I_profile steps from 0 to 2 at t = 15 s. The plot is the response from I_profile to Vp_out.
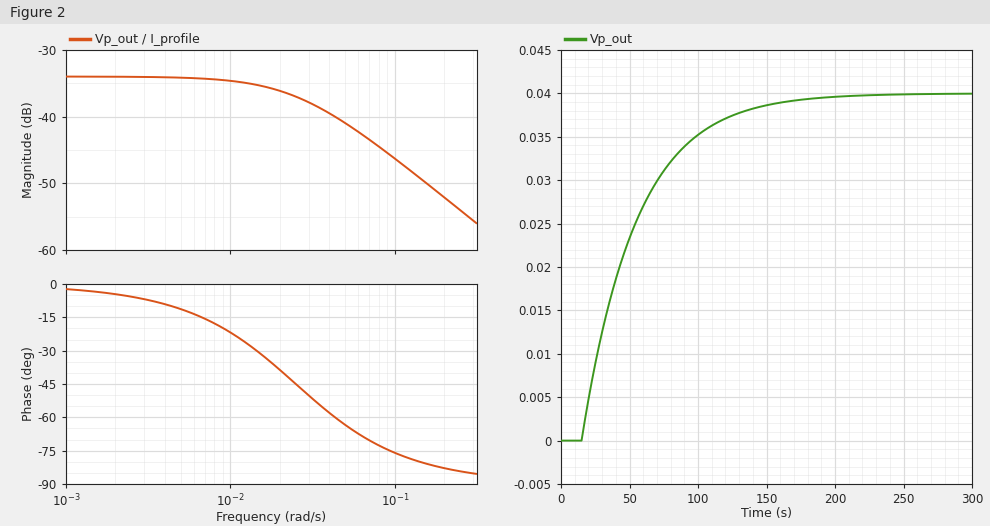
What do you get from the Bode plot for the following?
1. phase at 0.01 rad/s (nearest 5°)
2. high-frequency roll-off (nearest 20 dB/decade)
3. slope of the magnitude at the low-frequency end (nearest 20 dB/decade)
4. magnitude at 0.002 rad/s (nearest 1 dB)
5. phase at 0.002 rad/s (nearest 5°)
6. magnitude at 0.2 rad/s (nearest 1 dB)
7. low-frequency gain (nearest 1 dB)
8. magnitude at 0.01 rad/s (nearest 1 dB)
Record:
-20°
-20 dB/decade
0 dB/decade
-34 dB
-5°
-52 dB
-34 dB
-35 dB
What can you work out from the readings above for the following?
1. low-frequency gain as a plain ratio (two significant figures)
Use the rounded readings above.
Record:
0.020
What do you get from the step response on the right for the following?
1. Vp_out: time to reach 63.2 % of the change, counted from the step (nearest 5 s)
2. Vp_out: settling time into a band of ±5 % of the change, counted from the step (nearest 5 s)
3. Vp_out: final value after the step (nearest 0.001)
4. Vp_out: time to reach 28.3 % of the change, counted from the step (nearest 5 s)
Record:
40 s
120 s
0.040
15 s
